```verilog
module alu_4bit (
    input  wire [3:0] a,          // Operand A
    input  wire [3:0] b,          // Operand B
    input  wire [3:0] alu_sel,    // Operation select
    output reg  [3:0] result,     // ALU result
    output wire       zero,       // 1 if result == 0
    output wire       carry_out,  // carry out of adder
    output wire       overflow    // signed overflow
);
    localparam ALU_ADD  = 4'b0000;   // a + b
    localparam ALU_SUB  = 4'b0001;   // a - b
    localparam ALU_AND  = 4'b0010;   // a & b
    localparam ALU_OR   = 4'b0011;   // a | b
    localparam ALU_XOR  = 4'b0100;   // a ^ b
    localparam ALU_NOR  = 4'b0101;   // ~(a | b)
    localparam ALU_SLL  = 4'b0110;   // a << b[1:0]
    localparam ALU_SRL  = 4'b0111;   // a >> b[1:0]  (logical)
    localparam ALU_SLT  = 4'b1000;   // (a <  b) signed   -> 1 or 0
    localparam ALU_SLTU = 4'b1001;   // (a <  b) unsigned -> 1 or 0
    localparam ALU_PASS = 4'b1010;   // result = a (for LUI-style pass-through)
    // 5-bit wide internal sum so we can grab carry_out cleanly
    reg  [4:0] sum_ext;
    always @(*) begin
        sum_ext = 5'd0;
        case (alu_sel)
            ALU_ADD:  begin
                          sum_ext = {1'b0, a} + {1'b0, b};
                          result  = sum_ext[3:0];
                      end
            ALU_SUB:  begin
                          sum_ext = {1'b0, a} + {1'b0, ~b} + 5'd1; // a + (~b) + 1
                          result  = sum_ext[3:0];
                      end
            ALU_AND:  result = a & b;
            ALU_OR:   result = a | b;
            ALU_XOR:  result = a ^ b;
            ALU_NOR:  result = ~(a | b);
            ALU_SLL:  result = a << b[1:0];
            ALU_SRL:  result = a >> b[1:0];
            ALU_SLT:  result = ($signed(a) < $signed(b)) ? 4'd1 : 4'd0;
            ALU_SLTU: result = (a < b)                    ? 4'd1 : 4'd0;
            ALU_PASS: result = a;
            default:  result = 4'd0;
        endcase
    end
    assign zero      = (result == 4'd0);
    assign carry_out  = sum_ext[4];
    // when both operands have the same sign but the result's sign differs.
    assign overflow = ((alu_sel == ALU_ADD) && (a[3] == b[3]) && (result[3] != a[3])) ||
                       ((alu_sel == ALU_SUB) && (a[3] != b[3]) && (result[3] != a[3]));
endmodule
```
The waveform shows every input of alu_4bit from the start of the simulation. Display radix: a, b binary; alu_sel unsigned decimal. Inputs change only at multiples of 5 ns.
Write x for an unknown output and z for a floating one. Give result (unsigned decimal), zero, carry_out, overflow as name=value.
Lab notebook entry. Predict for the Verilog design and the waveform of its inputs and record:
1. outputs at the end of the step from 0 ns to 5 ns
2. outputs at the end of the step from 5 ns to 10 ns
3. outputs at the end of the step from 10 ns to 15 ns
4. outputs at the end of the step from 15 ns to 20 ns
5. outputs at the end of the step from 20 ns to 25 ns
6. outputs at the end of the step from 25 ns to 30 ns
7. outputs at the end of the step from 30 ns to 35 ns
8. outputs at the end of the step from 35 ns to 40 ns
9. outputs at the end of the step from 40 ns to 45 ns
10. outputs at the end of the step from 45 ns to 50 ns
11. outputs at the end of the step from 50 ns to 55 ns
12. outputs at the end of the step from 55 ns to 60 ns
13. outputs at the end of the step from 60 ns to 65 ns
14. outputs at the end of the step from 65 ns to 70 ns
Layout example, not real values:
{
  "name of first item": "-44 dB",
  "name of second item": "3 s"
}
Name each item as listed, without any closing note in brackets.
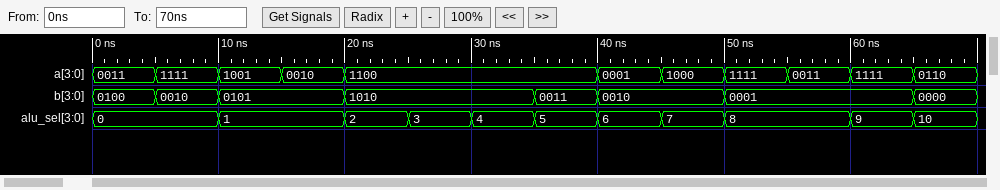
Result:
{
  "outputs at the end of the step from 0 ns to 5 ns": "result=7, zero=0, carry_out=0, overflow=0",
  "outputs at the end of the step from 5 ns to 10 ns": "result=1, zero=0, carry_out=1, overflow=0",
  "outputs at the end of the step from 10 ns to 15 ns": "result=4, zero=0, carry_out=1, overflow=1",
  "outputs at the end of the step from 15 ns to 20 ns": "result=13, zero=0, carry_out=0, overflow=0",
  "outputs at the end of the step from 20 ns to 25 ns": "result=8, zero=0, carry_out=0, overflow=0",
  "outputs at the end of the step from 25 ns to 30 ns": "result=14, zero=0, carry_out=0, overflow=0",
  "outputs at the end of the step from 30 ns to 35 ns": "result=6, zero=0, carry_out=0, overflow=0",
  "outputs at the end of the step from 35 ns to 40 ns": "result=0, zero=1, carry_out=0, overflow=0",
  "outputs at the end of the step from 40 ns to 45 ns": "result=4, zero=0, carry_out=0, overflow=0",
  "outputs at the end of the step from 45 ns to 50 ns": "result=2, zero=0, carry_out=0, overflow=0",
  "outputs at the end of the step from 50 ns to 55 ns": "result=1, zero=0, carry_out=0, overflow=0",
  "outputs at the end of the step from 55 ns to 60 ns": "result=0, zero=1, carry_out=0, overflow=0",
  "outputs at the end of the step from 60 ns to 65 ns": "result=0, zero=1, carry_out=0, overflow=0",
  "outputs at the end of the step from 65 ns to 70 ns": "result=6, zero=0, carry_out=0, overflow=0"
}
